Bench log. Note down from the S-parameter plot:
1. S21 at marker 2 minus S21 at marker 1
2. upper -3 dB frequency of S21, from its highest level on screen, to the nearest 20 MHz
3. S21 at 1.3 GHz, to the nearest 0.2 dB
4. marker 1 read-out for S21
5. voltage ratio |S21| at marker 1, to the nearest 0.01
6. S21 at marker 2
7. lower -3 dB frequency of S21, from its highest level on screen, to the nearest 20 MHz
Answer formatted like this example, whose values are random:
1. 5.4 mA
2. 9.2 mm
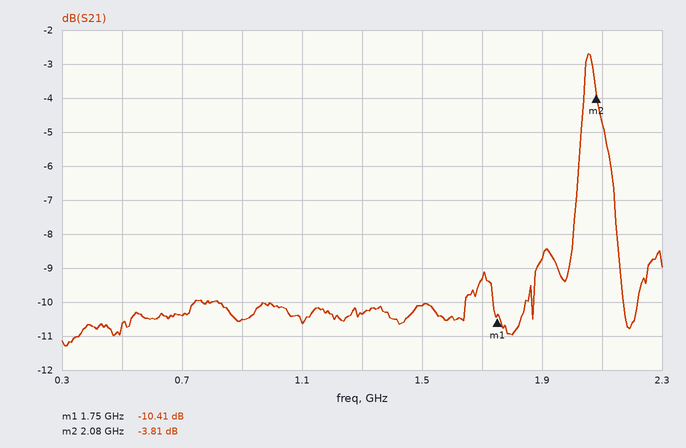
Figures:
1. 6.60 dB
2. 2.12 GHz
3. -10.4 dB
4. -10.41 dB
5. 0.30
6. -3.81 dB
7. 2.02 GHz
